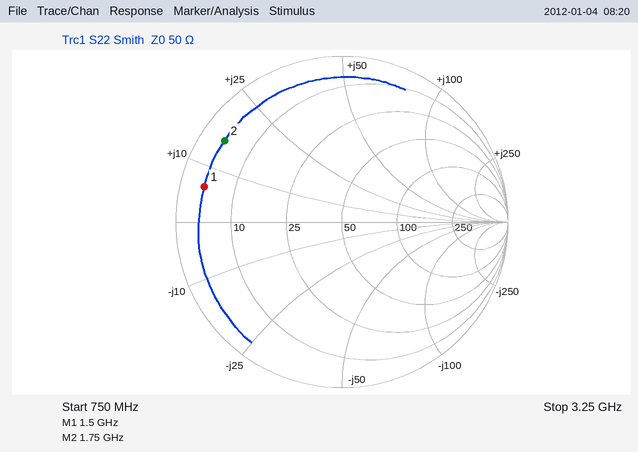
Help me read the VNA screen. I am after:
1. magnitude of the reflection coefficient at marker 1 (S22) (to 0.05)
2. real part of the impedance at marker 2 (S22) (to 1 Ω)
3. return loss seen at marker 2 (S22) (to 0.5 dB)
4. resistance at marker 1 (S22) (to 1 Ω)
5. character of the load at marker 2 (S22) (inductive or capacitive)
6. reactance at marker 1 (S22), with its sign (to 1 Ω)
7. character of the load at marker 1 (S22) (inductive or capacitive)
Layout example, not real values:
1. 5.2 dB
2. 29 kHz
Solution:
1. 0.85
2. 4 Ω
3. 1.5 dB
4. 4 Ω
5. inductive
6. +6 Ω
7. inductive
